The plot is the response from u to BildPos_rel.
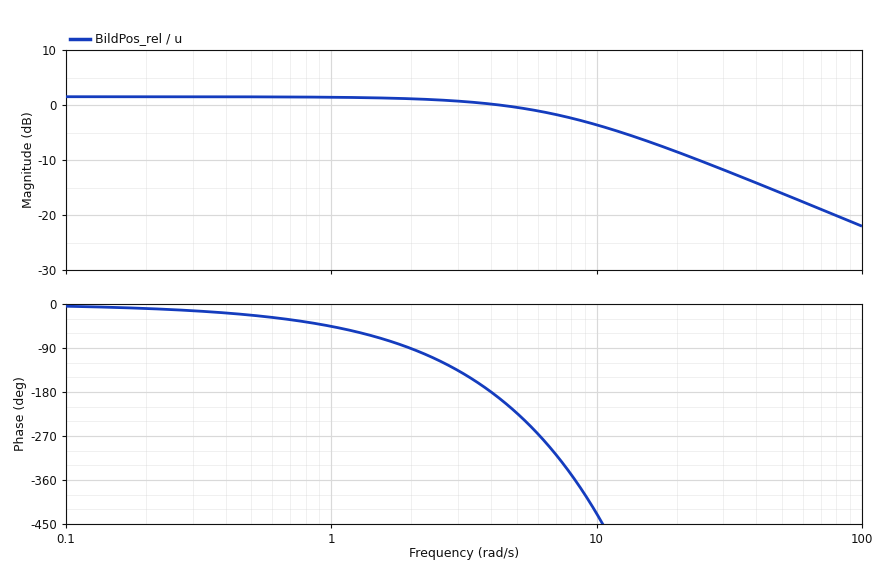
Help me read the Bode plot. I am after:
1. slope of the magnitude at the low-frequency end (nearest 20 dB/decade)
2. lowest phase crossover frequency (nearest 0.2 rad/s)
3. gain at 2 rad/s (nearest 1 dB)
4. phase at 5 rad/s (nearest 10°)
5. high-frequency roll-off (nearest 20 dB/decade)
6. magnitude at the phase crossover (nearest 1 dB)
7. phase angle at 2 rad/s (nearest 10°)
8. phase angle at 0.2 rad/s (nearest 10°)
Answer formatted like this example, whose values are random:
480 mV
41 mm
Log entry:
0 dB/decade
4.0 rad/s
1 dB
-220°
-20 dB/decade
0 dB
-90°
-10°
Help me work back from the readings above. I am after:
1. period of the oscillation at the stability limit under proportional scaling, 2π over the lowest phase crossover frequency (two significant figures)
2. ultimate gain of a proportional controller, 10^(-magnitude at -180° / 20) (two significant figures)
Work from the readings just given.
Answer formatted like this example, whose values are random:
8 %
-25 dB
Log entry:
1.6 s
1.0
